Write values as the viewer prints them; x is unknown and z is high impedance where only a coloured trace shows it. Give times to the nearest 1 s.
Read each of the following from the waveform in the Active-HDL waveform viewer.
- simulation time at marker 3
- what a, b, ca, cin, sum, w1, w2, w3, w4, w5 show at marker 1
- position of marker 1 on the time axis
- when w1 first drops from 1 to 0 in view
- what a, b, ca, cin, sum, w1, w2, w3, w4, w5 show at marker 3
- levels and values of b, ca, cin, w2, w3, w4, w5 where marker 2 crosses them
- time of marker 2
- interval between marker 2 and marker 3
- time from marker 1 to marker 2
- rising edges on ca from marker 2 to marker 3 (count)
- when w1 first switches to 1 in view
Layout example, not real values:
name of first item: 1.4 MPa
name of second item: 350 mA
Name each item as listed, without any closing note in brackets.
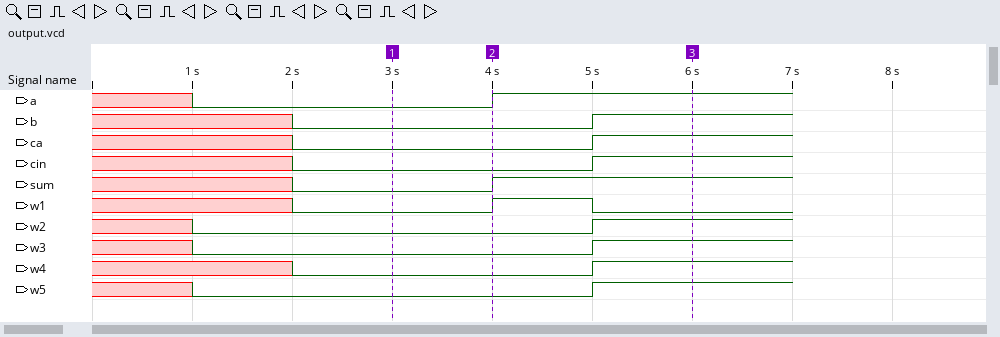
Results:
simulation time at marker 3: 6 s
what a, b, ca, cin, sum, w1, w2, w3, w4, w5 show at marker 1: a=0, b=0, ca=0, cin=0, sum=0, w1=0, w2=0, w3=0, w4=0, w5=0
position of marker 1 on the time axis: 3 s
when w1 first drops from 1 to 0 in view: 5 s
what a, b, ca, cin, sum, w1, w2, w3, w4, w5 show at marker 3: a=1, b=1, ca=1, cin=1, sum=1, w1=0, w2=1, w3=1, w4=1, w5=1
levels and values of b, ca, cin, w2, w3, w4, w5 where marker 2 crosses them: b=0, ca=0, cin=0, w2=0, w3=0, w4=0, w5=0
time of marker 2: 4 s
interval between marker 2 and marker 3: 2 s
time from marker 1 to marker 2: 1 s
rising edges on ca from marker 2 to marker 3: 1
when w1 first switches to 1 in view: 4 s
